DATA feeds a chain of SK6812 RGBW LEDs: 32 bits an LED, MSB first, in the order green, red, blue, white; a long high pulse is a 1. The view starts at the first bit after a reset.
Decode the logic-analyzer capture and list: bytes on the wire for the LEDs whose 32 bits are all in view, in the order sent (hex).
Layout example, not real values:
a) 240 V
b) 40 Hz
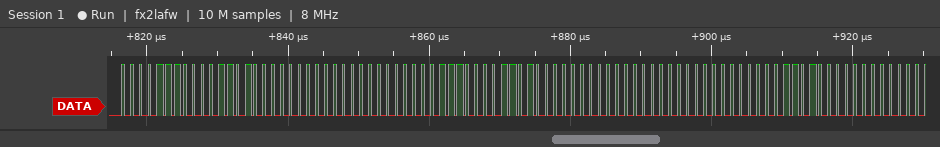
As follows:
a) 0E 1A 00 00 0E 1A 00 00
